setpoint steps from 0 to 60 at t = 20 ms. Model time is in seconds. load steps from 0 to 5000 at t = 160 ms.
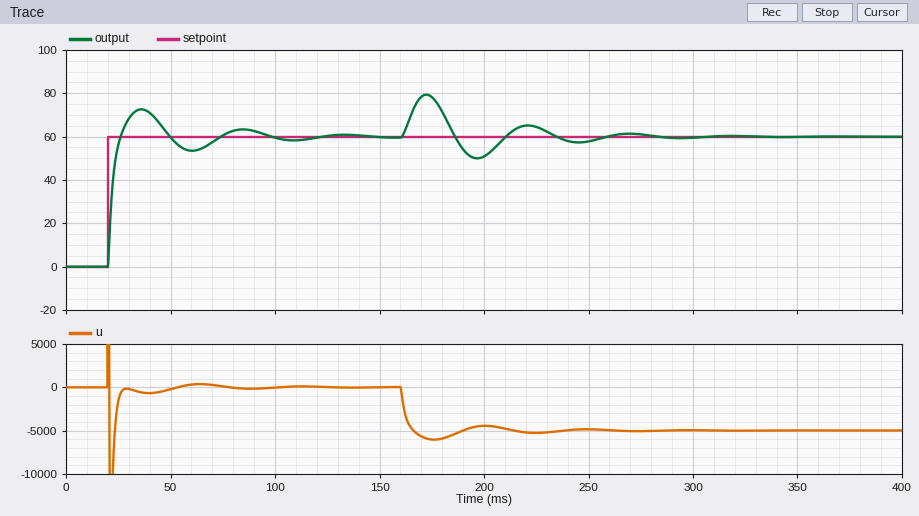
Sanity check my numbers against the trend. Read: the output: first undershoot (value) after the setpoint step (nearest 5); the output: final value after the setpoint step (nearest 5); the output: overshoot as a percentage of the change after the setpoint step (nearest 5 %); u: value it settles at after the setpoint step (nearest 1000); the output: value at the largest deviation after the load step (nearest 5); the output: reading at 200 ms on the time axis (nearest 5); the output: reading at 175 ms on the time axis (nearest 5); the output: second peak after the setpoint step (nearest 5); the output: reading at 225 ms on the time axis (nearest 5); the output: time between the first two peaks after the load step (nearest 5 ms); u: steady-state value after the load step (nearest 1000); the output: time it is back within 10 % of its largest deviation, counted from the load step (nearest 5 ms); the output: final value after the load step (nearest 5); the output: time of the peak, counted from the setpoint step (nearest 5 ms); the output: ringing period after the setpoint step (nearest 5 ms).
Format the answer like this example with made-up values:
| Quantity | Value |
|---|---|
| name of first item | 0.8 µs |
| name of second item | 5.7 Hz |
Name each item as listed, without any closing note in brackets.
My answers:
| Quantity | Value |
|---|---|
| the output: first undershoot (value) after the setpoint step | 55 |
| the output: final value after the setpoint step | 60 |
| the output: overshoot as a percentage of the change after the setpoint step | 20 % |
| u: value it settles at after the setpoint step | 0 |
| the output: value at the largest deviation after the load step | 80 |
| the output: reading at 200 ms on the time axis | 50 |
| the output: reading at 175 ms on the time axis | 80 |
| the output: second peak after the setpoint step | 65 |
| the output: reading at 225 ms on the time axis | 65 |
| the output: time between the first two peaks after the load step | 50 ms |
| u: steady-state value after the load step | -5000 |
| the output: time it is back within 10 % of its largest deviation, counted from the load step | 90 ms |
| the output: final value after the load step | 60 |
| the output: time of the peak, counted from the setpoint step | 15 ms |
| the output: ringing period after the setpoint step | 50 ms |
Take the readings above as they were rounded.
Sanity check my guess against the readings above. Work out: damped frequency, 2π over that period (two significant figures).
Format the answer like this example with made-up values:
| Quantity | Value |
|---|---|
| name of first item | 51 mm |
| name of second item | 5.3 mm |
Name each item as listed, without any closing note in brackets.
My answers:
| Quantity | Value |
|---|---|
| damped frequency, 2π over that period | 0.13 rad/ms |
